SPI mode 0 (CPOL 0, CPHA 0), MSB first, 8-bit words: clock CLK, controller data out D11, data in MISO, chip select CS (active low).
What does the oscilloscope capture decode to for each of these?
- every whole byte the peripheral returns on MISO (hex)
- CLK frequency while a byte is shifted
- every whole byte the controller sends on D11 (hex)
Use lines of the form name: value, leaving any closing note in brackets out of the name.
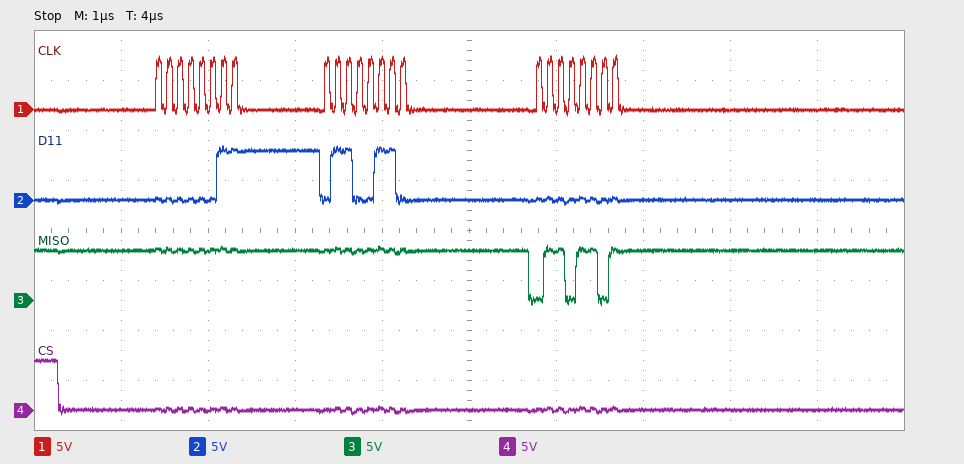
every whole byte the peripheral returns on MISO: FF FF 6D
CLK frequency while a byte is shifted: 8 MHz
every whole byte the controller sends on D11: 03 66 00
